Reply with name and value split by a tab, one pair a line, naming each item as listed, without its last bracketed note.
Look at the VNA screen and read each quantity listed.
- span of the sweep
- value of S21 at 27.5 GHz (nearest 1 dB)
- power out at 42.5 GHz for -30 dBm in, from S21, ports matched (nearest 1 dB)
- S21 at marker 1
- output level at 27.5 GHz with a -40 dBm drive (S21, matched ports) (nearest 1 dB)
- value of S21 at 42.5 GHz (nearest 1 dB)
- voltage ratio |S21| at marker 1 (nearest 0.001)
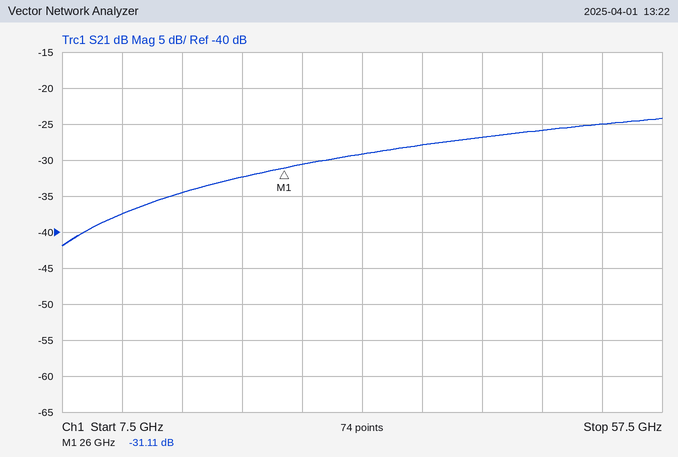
span of the sweep	50 GHz
value of S21 at 27.5 GHz	-31 dB
power out at 42.5 GHz for -30 dBm in, from S21, ports matched	-57 dBm
S21 at marker 1	-31.11 dB
output level at 27.5 GHz with a -40 dBm drive (S21, matched ports)	-71 dBm
value of S21 at 42.5 GHz	-27 dB
voltage ratio |S21| at marker 1	0.028
